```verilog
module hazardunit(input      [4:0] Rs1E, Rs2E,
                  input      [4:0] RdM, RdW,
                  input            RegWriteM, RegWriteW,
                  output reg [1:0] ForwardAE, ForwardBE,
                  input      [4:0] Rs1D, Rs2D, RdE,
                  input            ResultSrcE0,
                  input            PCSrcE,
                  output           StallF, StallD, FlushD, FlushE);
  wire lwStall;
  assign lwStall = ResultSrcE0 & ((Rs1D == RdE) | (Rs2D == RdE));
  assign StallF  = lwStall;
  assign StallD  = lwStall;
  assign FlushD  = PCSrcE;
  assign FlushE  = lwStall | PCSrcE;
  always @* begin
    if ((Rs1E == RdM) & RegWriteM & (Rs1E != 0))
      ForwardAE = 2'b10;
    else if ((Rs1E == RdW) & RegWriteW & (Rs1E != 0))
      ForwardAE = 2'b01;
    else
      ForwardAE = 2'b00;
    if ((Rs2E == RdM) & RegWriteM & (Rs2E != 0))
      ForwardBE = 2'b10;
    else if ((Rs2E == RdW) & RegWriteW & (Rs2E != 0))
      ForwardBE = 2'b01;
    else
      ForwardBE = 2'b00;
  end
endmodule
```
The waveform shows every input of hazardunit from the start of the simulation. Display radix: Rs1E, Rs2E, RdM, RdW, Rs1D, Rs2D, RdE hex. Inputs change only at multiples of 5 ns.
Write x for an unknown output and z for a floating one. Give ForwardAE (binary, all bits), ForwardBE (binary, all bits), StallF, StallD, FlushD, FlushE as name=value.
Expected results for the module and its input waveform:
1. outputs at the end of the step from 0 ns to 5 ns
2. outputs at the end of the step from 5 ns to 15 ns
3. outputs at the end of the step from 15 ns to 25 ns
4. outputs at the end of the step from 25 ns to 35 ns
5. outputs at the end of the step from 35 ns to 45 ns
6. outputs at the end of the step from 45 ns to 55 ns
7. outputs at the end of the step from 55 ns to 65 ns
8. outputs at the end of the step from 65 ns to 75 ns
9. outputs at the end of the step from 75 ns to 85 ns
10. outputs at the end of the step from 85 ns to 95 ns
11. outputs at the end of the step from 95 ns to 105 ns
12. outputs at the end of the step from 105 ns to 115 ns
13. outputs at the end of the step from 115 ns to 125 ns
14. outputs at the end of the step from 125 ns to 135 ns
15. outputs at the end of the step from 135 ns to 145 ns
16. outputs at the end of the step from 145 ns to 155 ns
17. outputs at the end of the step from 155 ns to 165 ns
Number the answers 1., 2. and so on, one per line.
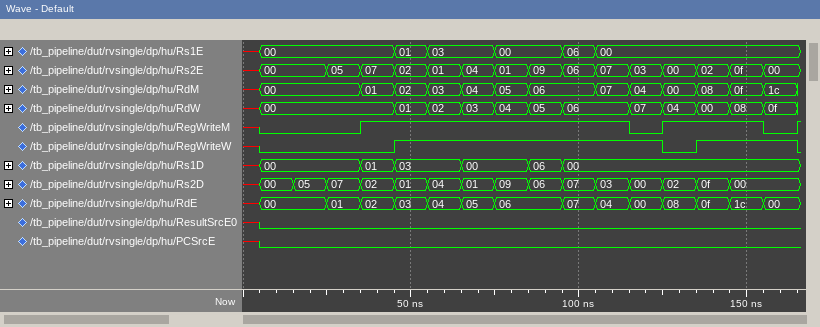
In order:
1. ForwardAE=x, ForwardBE=x, StallF=x, StallD=x, FlushD=x, FlushE=x
2. ForwardAE=00, ForwardBE=00, StallF=0, StallD=0, FlushD=0, FlushE=0
3. ForwardAE=00, ForwardBE=00, StallF=0, StallD=0, FlushD=0, FlushE=0
4. ForwardAE=00, ForwardBE=00, StallF=0, StallD=0, FlushD=0, FlushE=0
5. ForwardAE=00, ForwardBE=00, StallF=0, StallD=0, FlushD=0, FlushE=0
6. ForwardAE=01, ForwardBE=10, StallF=0, StallD=0, FlushD=0, FlushE=0
7. ForwardAE=10, ForwardBE=00, StallF=0, StallD=0, FlushD=0, FlushE=0
8. ForwardAE=01, ForwardBE=10, StallF=0, StallD=0, FlushD=0, FlushE=0
9. ForwardAE=00, ForwardBE=00, StallF=0, StallD=0, FlushD=0, FlushE=0
10. ForwardAE=00, ForwardBE=00, StallF=0, StallD=0, FlushD=0, FlushE=0
11. ForwardAE=10, ForwardBE=10, StallF=0, StallD=0, FlushD=0, FlushE=0
12. ForwardAE=00, ForwardBE=10, StallF=0, StallD=0, FlushD=0, FlushE=0
13. ForwardAE=00, ForwardBE=00, StallF=0, StallD=0, FlushD=0, FlushE=0
14. ForwardAE=00, ForwardBE=00, StallF=0, StallD=0, FlushD=0, FlushE=0
15. ForwardAE=00, ForwardBE=00, StallF=0, StallD=0, FlushD=0, FlushE=0
16. ForwardAE=00, ForwardBE=10, StallF=0, StallD=0, FlushD=0, FlushE=0
17. ForwardAE=00, ForwardBE=00, StallF=0, StallD=0, FlushD=0, FlushE=0
